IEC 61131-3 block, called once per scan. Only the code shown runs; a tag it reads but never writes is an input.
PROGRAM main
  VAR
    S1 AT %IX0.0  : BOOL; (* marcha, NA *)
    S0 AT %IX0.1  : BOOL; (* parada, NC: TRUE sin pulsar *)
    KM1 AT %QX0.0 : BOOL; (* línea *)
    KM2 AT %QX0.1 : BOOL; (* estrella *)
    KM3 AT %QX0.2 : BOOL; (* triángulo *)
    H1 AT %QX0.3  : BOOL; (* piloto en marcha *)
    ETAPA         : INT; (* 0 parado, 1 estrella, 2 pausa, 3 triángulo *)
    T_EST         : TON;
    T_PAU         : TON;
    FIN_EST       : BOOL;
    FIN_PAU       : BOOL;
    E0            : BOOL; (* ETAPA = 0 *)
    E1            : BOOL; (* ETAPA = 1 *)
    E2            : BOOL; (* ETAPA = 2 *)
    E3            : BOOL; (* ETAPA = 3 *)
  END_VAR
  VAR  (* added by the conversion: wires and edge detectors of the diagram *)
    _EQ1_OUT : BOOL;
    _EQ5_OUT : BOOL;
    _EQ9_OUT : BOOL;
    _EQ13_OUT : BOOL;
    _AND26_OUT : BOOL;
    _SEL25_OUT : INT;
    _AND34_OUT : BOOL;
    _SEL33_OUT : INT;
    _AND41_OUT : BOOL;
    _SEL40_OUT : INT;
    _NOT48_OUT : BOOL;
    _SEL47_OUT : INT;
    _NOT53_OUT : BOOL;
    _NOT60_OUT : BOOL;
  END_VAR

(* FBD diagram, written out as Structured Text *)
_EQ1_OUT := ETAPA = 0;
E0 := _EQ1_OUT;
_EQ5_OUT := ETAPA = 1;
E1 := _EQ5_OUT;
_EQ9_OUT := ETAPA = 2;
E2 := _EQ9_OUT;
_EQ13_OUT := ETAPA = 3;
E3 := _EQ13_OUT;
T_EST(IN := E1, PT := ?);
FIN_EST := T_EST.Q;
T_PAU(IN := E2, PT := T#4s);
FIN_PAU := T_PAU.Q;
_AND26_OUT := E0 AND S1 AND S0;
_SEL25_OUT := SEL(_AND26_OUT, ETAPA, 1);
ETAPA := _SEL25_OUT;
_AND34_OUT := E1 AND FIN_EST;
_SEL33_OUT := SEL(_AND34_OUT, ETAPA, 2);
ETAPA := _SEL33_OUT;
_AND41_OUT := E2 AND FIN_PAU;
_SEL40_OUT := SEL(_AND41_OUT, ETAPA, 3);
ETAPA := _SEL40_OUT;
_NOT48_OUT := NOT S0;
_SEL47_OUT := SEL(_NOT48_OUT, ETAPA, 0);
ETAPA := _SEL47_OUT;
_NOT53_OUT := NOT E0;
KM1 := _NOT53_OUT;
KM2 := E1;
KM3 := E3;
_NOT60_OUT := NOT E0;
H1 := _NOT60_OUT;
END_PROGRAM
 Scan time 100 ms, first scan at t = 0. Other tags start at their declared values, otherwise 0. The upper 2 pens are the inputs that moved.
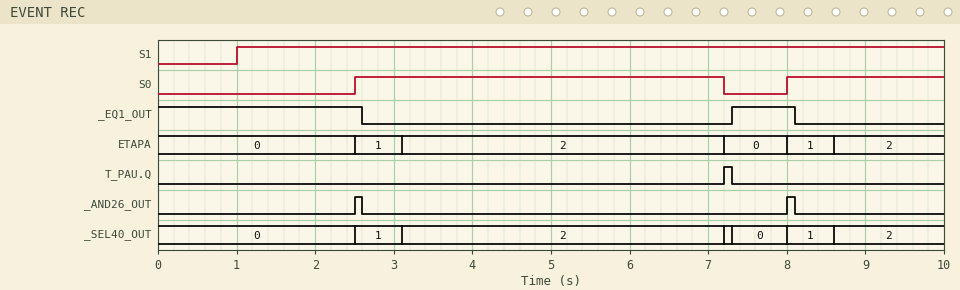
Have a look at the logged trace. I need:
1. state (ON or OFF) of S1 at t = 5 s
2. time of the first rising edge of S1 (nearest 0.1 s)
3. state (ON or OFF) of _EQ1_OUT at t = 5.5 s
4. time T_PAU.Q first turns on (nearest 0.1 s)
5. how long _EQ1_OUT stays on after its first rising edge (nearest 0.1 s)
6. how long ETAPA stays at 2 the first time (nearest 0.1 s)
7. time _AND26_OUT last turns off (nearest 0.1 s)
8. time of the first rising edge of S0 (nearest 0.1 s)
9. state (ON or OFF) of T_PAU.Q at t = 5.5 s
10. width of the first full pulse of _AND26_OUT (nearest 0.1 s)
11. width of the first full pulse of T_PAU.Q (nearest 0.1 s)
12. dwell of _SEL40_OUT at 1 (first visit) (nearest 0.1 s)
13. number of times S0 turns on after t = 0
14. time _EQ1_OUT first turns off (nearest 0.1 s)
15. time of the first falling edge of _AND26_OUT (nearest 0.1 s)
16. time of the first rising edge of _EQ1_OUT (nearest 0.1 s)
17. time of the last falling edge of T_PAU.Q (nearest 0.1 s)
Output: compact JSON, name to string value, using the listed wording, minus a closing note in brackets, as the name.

{"state (ON or OFF) of S1 at t = 5 s": "ON", "time of the first rising edge of S1": "1.0 s", "state (ON or OFF) of _EQ1_OUT at t = 5.5 s": "OFF", "time T_PAU.Q first turns on": "7.2 s", "how long _EQ1_OUT stays on after its first rising edge": "0.8 s", "how long ETAPA stays at 2 the first time": "4.1 s", "time _AND26_OUT last turns off": "8.1 s", "time of the first rising edge of S0": "2.5 s", "state (ON or OFF) of T_PAU.Q at t = 5.5 s": "OFF", "width of the first full pulse of _AND26_OUT": "0.1 s", "width of the first full pulse of T_PAU.Q": "0.1 s", "dwell of _SEL40_OUT at 1 (first visit)": "0.6 s", "number of times S0 turns on after t = 0": "2", "time _EQ1_OUT first turns off": "2.6 s", "time of the first falling edge of _AND26_OUT": "2.6 s", "time of the first rising edge of _EQ1_OUT": "7.3 s", "time of the last falling edge of T_PAU.Q": "7.3 s"}
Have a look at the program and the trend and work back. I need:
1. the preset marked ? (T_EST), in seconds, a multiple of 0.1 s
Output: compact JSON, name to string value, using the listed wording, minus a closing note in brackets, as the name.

{"the preset marked ? (T_EST), in seconds, a multiple of 0.1 s": "0.5 s"}
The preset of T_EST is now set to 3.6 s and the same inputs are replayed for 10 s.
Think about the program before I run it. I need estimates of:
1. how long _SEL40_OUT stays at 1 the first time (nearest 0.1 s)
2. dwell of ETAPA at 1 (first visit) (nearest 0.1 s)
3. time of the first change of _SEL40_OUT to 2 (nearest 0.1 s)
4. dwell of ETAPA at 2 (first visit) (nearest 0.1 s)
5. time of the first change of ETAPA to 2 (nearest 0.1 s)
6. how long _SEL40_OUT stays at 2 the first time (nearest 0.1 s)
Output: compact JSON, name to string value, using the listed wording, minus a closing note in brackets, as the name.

{"how long _SEL40_OUT stays at 1 the first time": "3.7 s", "dwell of ETAPA at 1 (first visit)": "3.7 s", "time of the first change of _SEL40_OUT to 2": "6.2 s", "dwell of ETAPA at 2 (first visit)": "1.0 s", "time of the first change of ETAPA to 2": "6.2 s", "how long _SEL40_OUT stays at 2 the first time": "1.1 s"}
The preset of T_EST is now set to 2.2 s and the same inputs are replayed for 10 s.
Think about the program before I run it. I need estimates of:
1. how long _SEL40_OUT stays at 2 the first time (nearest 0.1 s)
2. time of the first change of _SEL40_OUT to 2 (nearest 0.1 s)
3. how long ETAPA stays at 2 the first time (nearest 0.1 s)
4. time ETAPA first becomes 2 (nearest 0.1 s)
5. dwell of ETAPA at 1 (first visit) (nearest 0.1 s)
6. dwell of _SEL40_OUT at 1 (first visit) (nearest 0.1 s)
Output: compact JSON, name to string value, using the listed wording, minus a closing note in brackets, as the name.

{"how long _SEL40_OUT stays at 2 the first time": "2.5 s", "time of the first change of _SEL40_OUT to 2": "4.8 s", "how long ETAPA stays at 2 the first time": "2.4 s", "time ETAPA first becomes 2": "4.8 s", "dwell of ETAPA at 1 (first visit)": "2.3 s", "dwell of _SEL40_OUT at 1 (first visit)": "2.3 s"}
